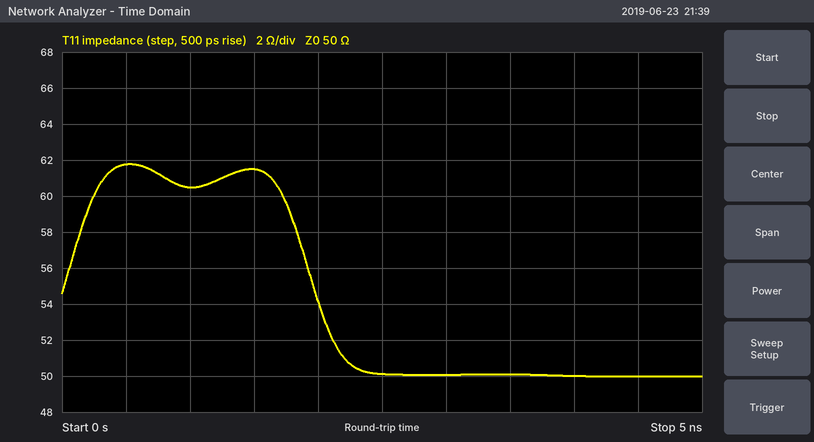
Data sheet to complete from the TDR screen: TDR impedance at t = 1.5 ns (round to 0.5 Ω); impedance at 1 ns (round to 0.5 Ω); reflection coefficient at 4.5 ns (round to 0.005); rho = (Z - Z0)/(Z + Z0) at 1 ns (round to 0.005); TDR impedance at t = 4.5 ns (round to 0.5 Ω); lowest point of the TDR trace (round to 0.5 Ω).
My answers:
61.5 Ω
60.5 Ω
0.000
+0.095
50.0 Ω
50.0 Ω
